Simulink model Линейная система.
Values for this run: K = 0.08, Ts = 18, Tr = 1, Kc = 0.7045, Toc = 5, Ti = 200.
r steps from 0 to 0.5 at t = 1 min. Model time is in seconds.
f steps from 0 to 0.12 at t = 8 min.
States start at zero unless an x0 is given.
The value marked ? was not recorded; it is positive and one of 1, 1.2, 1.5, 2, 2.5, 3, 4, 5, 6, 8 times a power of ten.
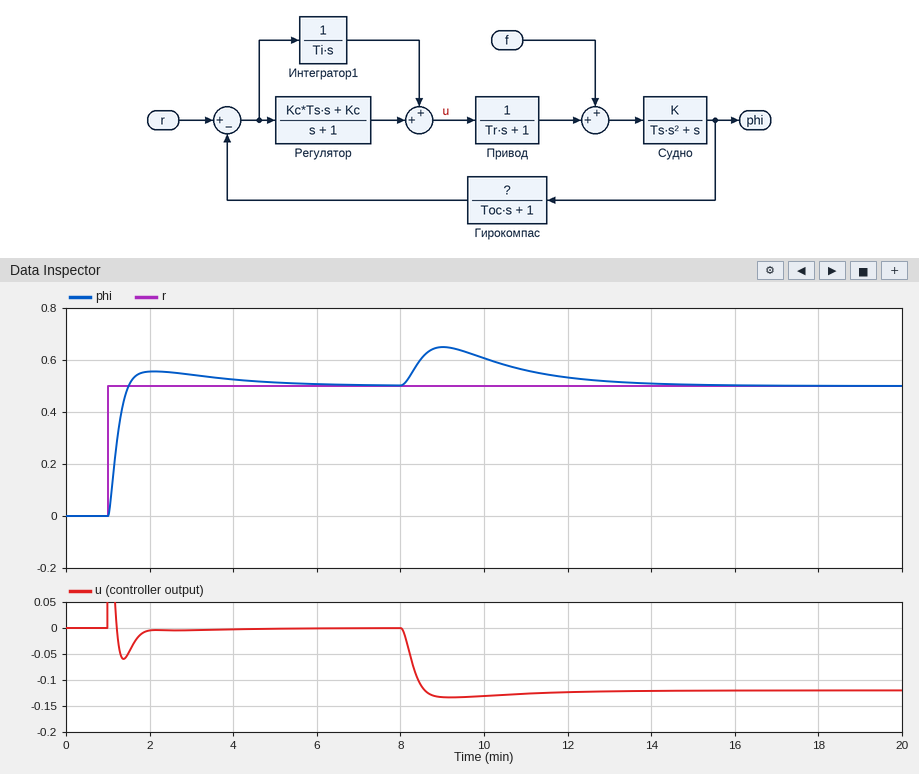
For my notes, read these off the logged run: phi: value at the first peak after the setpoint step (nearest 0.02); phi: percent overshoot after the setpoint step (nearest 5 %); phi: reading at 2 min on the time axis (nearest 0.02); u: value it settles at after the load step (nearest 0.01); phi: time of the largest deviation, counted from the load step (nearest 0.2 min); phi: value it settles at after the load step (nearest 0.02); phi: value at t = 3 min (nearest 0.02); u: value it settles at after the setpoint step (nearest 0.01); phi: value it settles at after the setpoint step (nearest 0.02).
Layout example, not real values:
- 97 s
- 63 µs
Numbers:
- 0.56
- 10 %
- 0.56
- -0.12
- 1.0 min
- 0.50
- 0.54
- 0.00
- 0.50
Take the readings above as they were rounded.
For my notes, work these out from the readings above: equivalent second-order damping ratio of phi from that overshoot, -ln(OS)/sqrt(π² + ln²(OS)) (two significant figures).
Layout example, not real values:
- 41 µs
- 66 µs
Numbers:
- 0.59
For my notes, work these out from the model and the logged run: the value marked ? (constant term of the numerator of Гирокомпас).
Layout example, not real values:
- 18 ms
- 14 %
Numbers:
- 1
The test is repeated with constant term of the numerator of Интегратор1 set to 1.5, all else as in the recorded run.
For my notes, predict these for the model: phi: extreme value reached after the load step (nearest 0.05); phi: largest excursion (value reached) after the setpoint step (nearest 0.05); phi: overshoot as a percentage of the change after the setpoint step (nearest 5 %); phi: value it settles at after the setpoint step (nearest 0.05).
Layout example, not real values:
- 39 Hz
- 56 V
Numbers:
- 0.65
- 0.60
- 15 %
- 0.50
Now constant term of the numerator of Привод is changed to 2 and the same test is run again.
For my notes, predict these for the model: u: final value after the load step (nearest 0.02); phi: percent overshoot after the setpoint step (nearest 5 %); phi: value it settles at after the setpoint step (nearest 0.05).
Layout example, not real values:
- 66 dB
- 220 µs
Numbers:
- -0.06
- 25 %
- 0.50
